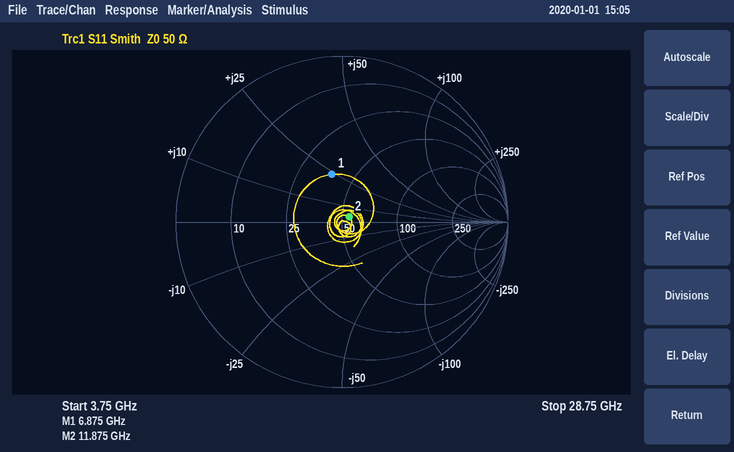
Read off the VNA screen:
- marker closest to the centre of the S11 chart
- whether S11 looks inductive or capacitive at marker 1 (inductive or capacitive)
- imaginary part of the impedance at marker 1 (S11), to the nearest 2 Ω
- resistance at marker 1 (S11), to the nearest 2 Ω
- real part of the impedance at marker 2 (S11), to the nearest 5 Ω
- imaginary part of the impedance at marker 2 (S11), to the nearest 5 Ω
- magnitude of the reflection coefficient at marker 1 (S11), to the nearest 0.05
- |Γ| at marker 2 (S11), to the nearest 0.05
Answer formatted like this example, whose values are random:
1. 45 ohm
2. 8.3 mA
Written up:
1. marker 2
2. inductive
3. +24 Ω
4. 38 Ω
5. 55 Ω
6. +5 Ω
7. 0.30
8. 0.05
